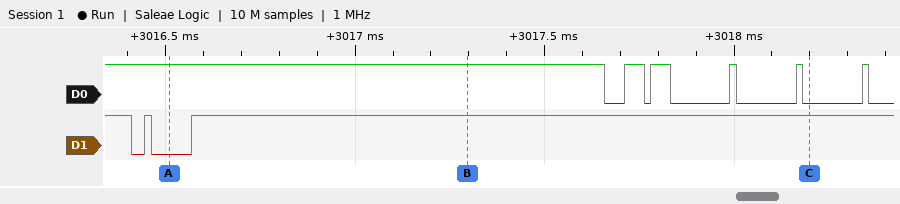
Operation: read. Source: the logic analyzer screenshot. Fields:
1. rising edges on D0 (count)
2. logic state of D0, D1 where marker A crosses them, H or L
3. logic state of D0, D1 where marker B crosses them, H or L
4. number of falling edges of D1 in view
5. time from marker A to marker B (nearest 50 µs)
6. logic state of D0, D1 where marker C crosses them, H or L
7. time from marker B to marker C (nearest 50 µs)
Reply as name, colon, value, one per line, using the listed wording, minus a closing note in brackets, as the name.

rising edges on D0: 5
logic state of D0, D1 where marker A crosses them, H or L: D0=H, D1=L
logic state of D0, D1 where marker B crosses them, H or L: D0=H, D1=H
number of falling edges of D1 in view: 2
time from marker A to marker B: 800 µs
logic state of D0, D1 where marker C crosses them, H or L: D0=L, D1=H
time from marker B to marker C: 900 µs
